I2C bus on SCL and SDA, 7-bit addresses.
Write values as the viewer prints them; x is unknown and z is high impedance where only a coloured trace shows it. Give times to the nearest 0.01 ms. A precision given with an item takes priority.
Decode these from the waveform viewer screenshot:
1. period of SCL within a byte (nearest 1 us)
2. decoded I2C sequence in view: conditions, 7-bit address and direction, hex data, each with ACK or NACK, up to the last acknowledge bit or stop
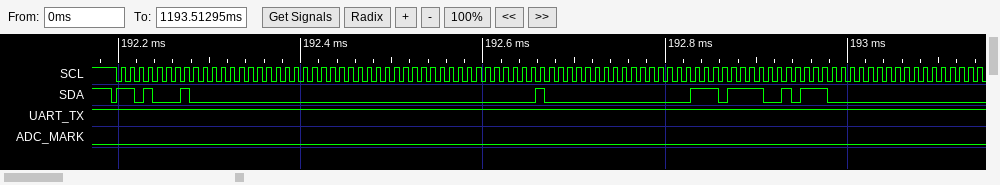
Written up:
10 us
start, address 68 read ACK, 00 ACK, 00 ACK, 00 ACK, 00 ACK, 40 ACK, 00 ACK, EF ACK, 5C ACK, 00 ACK
